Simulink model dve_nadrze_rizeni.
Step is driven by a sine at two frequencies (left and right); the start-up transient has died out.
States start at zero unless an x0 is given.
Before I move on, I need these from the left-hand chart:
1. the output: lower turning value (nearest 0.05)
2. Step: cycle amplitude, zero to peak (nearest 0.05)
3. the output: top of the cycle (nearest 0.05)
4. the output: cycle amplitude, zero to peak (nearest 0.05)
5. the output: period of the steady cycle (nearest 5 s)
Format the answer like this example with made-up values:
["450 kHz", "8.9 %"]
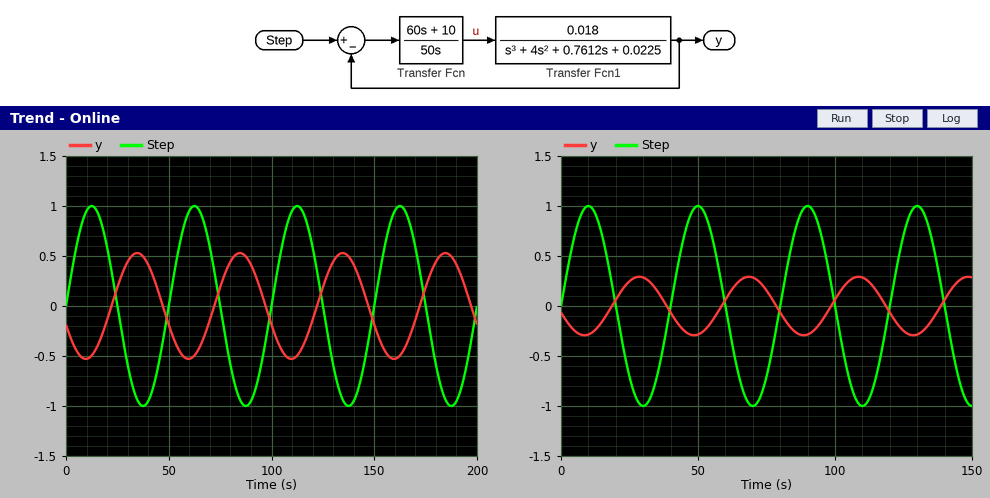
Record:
["-0.55", "1.00", "0.55", "0.55", "50 s"]
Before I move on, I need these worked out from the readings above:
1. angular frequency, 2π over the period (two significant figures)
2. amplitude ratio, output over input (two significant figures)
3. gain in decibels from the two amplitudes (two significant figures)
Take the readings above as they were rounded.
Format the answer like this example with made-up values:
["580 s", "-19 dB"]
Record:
["0.13 rad/s", "0.55", "-5.2 dB"]
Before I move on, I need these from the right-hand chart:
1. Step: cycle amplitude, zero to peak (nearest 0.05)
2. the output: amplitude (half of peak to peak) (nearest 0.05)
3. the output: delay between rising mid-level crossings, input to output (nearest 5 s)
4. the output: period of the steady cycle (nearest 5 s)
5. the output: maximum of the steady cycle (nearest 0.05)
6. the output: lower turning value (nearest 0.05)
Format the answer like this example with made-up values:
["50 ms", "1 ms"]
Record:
["1.00", "0.30", "20 s", "40 s", "0.30", "-0.30"]
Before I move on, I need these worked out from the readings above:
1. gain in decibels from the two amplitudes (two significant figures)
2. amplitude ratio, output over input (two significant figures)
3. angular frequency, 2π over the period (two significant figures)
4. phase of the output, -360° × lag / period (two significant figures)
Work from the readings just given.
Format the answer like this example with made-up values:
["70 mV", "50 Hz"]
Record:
["-10 dB", "0.30", "0.16 rad/s", "-180°"]
